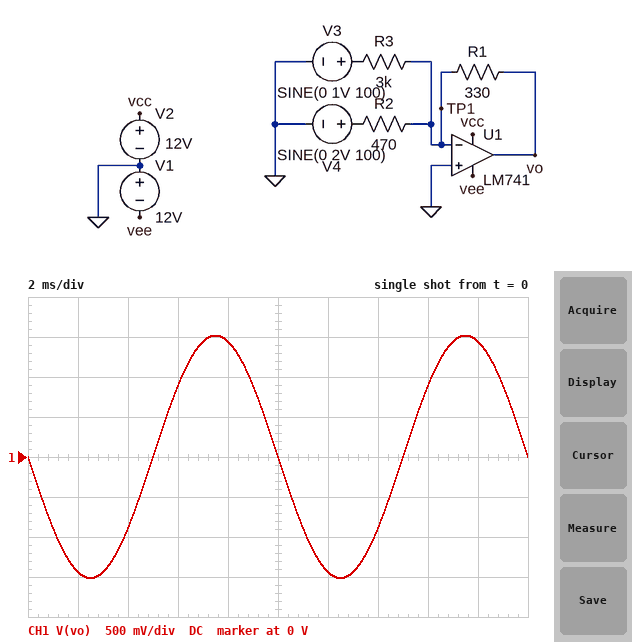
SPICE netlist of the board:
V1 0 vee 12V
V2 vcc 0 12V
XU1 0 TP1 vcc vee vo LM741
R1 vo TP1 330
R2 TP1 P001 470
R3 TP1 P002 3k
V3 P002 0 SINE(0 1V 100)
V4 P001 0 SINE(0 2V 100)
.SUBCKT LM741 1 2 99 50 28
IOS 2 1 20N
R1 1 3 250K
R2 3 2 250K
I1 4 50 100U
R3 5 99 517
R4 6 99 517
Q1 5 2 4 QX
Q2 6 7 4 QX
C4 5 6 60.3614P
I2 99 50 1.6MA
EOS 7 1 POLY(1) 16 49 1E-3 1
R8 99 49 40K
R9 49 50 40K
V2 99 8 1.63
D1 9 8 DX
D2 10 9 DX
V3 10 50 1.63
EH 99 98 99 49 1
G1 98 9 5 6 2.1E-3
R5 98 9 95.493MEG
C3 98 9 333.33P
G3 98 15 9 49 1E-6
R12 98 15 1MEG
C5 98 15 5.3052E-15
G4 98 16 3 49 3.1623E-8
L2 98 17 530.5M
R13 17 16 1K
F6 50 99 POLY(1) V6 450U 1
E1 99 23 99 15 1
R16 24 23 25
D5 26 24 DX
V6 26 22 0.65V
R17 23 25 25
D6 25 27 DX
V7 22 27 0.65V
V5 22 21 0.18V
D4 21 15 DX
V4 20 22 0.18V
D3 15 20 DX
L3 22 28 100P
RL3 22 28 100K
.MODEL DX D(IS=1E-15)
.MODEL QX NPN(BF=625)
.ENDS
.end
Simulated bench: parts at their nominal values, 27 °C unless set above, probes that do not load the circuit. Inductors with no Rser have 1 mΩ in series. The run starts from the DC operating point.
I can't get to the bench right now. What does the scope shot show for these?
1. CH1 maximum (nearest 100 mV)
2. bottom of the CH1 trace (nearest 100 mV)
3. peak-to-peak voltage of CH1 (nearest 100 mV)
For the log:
1.5 V
-1.5 V
3.0 V
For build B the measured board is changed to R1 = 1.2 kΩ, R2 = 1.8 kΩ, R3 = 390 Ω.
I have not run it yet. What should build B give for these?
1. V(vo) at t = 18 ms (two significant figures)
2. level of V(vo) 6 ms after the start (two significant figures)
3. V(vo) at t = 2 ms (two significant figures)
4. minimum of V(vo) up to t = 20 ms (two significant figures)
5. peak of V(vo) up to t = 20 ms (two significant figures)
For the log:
4.2 V
2.6 V
-4.2 V
-4.4 V
4.4 V
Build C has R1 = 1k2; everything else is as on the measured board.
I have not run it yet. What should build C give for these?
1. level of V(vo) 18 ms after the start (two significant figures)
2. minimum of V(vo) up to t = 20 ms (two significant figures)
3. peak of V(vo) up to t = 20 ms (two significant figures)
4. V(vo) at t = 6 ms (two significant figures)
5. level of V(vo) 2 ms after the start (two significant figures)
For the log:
5.2 V
-5.5 V
5.5 V
3.2 V
-5.2 V
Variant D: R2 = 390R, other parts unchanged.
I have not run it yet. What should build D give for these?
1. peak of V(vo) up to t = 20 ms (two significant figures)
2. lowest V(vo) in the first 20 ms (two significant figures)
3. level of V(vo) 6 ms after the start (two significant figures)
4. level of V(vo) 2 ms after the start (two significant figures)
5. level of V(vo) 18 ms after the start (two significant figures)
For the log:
1.8 V
-1.8 V
1.1 V
-1.7 V
1.7 V
